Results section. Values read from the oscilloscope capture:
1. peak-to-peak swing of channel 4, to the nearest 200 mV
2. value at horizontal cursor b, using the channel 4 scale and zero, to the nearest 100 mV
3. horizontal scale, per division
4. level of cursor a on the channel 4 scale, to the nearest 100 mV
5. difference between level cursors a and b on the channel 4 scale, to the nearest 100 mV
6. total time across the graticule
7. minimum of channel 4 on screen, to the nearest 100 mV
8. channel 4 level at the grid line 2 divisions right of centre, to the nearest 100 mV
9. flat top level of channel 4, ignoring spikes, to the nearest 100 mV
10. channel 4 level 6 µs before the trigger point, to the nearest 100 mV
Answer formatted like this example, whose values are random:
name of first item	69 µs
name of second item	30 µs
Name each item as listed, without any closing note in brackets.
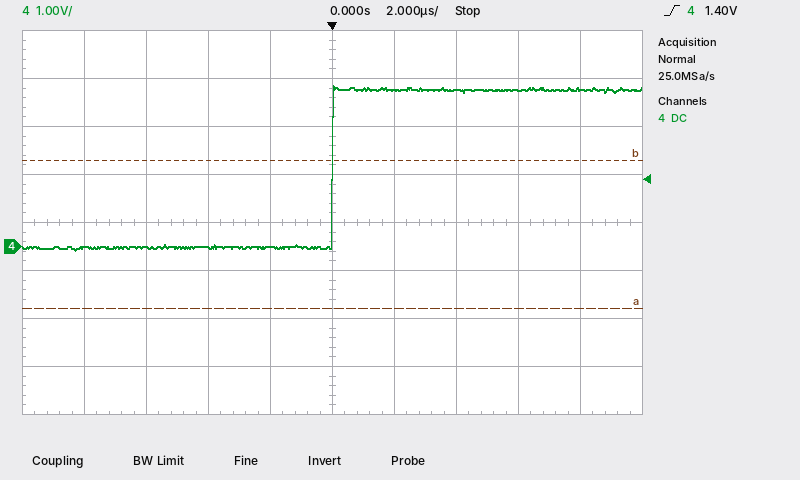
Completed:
peak-to-peak swing of channel 4, to the nearest 200 mV	3.4 V
value at horizontal cursor b, using the channel 4 scale and zero, to the nearest 100 mV	1.8 V
horizontal scale, per division	2 µs
level of cursor a on the channel 4 scale, to the nearest 100 mV	-1.3 V
difference between level cursors a and b on the channel 4 scale, to the nearest 100 mV	3.1 V
total time across the graticule	20 µs
minimum of channel 4 on screen, to the nearest 100 mV	-100 mV
channel 4 level at the grid line 2 divisions right of centre, to the nearest 100 mV	3.3 V
flat top level of channel 4, ignoring spikes, to the nearest 100 mV	3.3 V
channel 4 level 6 µs before the trigger point, to the nearest 100 mV	0.0 V
